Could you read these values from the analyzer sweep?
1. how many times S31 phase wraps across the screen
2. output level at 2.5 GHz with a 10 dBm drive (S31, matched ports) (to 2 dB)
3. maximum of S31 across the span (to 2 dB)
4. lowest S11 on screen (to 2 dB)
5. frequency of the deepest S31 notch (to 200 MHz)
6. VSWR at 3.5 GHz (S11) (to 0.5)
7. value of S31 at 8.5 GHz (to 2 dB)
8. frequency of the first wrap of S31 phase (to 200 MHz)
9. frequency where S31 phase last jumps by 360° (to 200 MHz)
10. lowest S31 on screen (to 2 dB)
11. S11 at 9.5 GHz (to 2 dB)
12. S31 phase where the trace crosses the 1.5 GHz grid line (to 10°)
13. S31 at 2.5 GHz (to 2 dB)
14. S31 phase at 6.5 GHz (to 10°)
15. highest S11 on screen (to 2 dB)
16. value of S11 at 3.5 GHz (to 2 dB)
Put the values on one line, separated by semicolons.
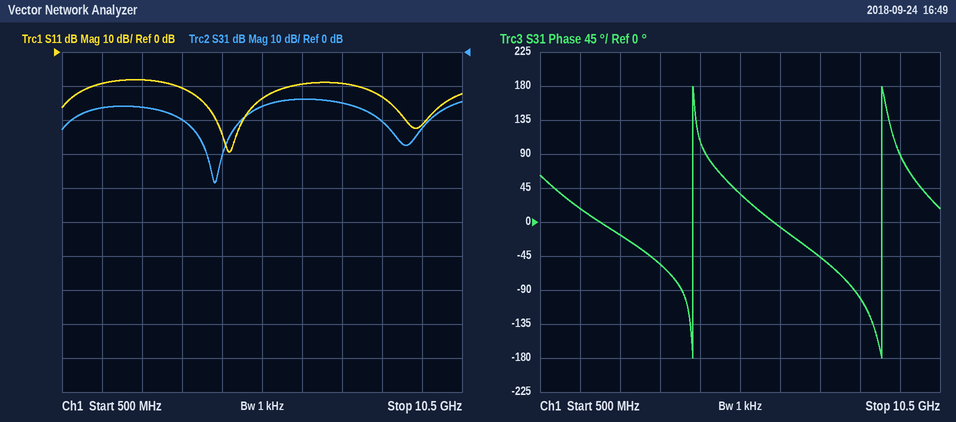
2; -6 dBm; -14 dB; -30 dB; 4.4 GHz; 2.0; -20 dB; 4.4 GHz; 9.0 GHz; -38 dB; -22 dB; 20°; -16 dB; -10°; -8 dB; -10 dB
